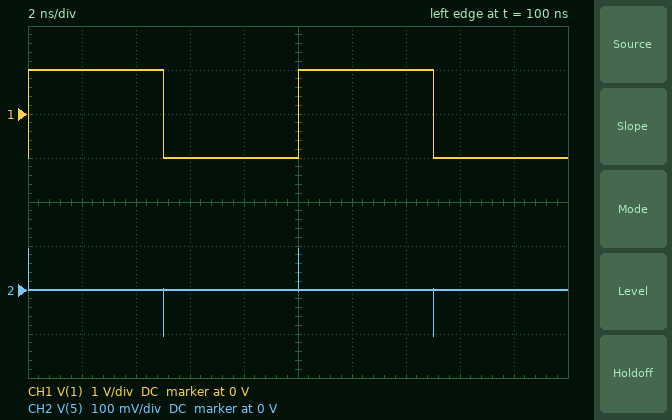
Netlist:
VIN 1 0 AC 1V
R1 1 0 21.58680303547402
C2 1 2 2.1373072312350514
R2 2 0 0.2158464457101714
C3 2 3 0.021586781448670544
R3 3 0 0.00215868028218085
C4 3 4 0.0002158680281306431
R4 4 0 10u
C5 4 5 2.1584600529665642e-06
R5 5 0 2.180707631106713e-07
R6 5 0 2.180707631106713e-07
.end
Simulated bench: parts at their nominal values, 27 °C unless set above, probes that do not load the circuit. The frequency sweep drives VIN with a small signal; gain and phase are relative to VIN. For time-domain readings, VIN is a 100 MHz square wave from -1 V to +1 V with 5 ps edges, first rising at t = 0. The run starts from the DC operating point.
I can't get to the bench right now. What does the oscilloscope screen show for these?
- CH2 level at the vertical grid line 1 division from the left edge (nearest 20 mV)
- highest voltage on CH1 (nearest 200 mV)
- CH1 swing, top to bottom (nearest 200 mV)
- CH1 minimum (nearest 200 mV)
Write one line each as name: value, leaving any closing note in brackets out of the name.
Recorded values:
CH2 level at the vertical grid line 1 division from the left edge: 0 V
highest voltage on CH1: 1.0 V
CH1 swing, top to bottom: 2.0 V
CH1 minimum: -1.0 V
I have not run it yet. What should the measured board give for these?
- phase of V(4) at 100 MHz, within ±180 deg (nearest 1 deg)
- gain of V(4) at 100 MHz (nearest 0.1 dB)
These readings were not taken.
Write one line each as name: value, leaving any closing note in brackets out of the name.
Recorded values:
phase of V(4) at 100 MHz, within ±180 deg: 36 deg
gain of V(4) at 100 MHz: -2.0 dB
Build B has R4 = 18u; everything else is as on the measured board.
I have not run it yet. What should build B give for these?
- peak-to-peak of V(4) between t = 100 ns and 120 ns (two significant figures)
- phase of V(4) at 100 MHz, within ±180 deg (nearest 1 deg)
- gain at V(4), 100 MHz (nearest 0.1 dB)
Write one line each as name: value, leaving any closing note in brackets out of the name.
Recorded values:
peak-to-peak of V(4) between t = 100 ns and 120 ns: 3.1 V
phase of V(4) at 100 MHz, within ±180 deg: 22 deg
gain at V(4), 100 MHz: -0.8 dB
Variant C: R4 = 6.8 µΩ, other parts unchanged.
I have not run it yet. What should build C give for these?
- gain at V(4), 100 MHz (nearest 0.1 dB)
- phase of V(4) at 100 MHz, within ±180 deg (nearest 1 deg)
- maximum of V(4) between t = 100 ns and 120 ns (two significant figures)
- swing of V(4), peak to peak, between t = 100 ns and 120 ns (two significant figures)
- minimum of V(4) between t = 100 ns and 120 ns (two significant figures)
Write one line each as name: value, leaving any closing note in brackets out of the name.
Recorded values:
gain at V(4), 100 MHz: -3.5 dB
phase of V(4) at 100 MHz, within ±180 deg: 47 deg
maximum of V(4) between t = 100 ns and 120 ns: 1.9 V
swing of V(4), peak to peak, between t = 100 ns and 120 ns: 3.8 V
minimum of V(4) between t = 100 ns and 120 ns: -1.9 V
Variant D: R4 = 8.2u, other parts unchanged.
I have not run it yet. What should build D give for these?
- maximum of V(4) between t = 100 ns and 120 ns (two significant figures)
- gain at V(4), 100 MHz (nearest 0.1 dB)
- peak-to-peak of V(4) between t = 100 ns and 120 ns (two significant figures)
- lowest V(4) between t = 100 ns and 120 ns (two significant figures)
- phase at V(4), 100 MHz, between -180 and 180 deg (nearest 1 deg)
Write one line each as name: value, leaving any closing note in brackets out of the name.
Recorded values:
maximum of V(4) between t = 100 ns and 120 ns: 1.9 V
gain at V(4), 100 MHz: -2.7 dB
peak-to-peak of V(4) between t = 100 ns and 120 ns: 3.7 V
lowest V(4) between t = 100 ns and 120 ns: -1.9 V
phase at V(4), 100 MHz, between -180 and 180 deg: 42 deg
